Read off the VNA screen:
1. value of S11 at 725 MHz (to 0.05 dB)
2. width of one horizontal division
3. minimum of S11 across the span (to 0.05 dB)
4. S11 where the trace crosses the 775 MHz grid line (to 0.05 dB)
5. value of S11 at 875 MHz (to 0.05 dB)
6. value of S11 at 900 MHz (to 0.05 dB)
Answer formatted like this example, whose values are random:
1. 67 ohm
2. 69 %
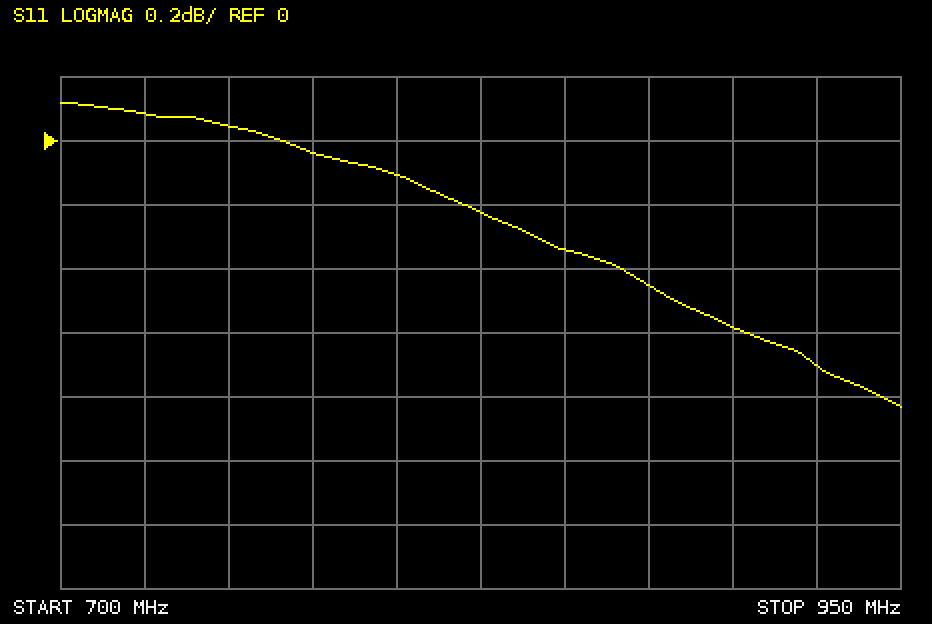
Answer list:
1. 0.10 dB
2. 25 MHz
3. -0.85 dB
4. -0.05 dB
5. -0.45 dB
6. -0.60 dB
